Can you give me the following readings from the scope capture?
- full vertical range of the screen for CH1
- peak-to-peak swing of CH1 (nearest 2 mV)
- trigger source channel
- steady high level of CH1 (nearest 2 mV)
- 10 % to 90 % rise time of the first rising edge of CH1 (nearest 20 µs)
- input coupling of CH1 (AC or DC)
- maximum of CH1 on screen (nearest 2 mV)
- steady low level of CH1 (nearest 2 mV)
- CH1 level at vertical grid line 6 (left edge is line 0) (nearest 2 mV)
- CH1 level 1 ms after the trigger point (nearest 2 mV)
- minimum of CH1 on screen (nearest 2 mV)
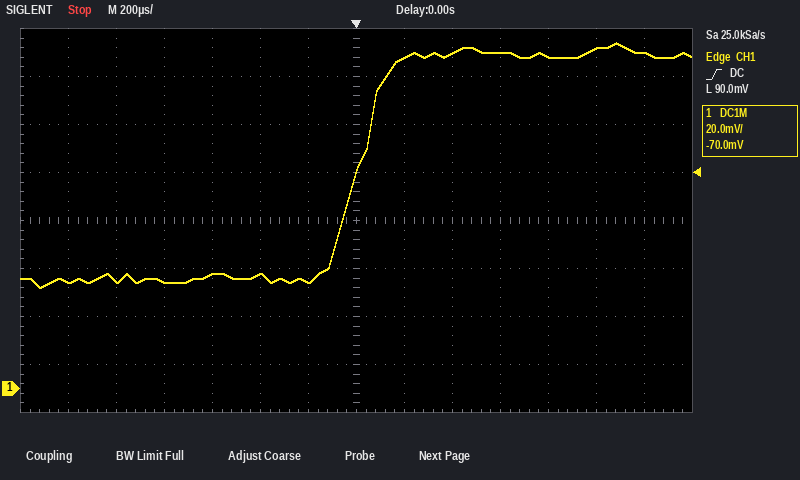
160 mV
102 mV
CH1
138 mV
220 µs
DC
144 mV
46 mV
44 mV
142 mV
42 mV
